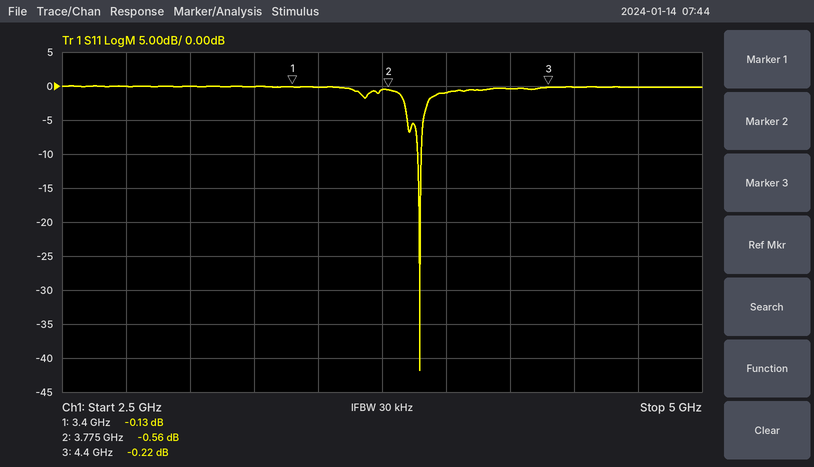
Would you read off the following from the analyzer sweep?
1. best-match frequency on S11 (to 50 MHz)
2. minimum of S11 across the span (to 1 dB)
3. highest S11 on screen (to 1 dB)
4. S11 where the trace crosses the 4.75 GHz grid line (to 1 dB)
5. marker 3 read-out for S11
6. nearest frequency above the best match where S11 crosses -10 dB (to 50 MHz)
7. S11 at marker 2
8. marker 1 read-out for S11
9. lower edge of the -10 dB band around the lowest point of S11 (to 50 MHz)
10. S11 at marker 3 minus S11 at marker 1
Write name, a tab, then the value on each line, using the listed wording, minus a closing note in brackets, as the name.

best-match frequency on S11	3.90 GHz
minimum of S11 across the span	-42 dB
highest S11 on screen	0 dB
S11 where the trace crosses the 4.75 GHz grid line	0 dB
marker 3 read-out for S11	-0.22 dB
nearest frequency above the best match where S11 crosses -10 dB	3.90 GHz
S11 at marker 2	-0.56 dB
marker 1 read-out for S11	-0.13 dB
lower edge of the -10 dB band around the lowest point of S11	3.90 GHz
S11 at marker 3 minus S11 at marker 1	-0.09 dB
